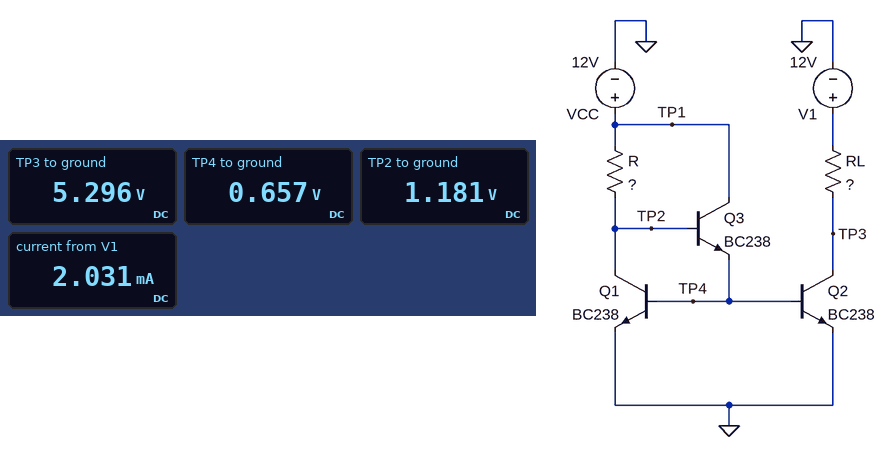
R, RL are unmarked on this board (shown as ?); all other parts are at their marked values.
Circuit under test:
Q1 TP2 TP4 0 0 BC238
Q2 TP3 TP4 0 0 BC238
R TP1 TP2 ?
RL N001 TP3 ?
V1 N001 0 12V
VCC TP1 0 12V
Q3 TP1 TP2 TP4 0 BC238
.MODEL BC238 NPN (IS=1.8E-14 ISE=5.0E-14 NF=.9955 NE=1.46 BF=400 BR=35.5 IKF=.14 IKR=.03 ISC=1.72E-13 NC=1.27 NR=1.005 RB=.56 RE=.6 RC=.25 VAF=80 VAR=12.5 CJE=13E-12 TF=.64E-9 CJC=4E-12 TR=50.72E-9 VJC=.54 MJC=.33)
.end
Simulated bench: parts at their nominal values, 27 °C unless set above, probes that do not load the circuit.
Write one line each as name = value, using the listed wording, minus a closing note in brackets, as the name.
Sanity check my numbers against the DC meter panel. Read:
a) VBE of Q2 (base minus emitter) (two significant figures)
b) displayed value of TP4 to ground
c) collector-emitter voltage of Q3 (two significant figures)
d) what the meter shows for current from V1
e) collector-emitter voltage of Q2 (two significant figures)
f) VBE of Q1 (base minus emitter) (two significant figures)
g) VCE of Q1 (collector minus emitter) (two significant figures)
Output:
VBE of Q2 (base minus emitter) = 660 mV
displayed value of TP4 to ground = 0.657 V
collector-emitter voltage of Q3 = 11 V
what the meter shows for current from V1 = 2.031 mA
collector-emitter voltage of Q2 = 5.3 V
VBE of Q1 (base minus emitter) = 660 mV
VCE of Q1 (collector minus emitter) = 1.2 V
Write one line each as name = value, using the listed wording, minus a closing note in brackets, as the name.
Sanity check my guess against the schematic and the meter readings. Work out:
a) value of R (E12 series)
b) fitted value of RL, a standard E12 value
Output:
value of R = 5.6 kΩ
fitted value of RL, a standard E12 value = 3.3 kΩ
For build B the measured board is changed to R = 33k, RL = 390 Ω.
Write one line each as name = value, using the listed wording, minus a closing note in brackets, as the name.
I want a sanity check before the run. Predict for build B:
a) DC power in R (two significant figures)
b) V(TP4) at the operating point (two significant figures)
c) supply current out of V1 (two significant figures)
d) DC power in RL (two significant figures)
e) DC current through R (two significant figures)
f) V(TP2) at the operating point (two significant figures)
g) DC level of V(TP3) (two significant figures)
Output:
DC power in R = 3.6 mW
V(TP4) at the operating point = 610 mV
supply current out of V1 = 380 µA
DC power in RL = 55 µW
DC current through R = 330 µA
V(TP2) at the operating point = 1.1 V
DC level of V(TP3) = 12 V
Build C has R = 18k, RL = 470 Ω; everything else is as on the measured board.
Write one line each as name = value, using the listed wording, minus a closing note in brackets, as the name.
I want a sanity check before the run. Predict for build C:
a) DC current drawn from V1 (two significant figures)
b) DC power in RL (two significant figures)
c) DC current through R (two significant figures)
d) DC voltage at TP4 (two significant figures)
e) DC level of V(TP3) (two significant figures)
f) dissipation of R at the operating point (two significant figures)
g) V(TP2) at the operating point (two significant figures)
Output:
DC current drawn from V1 = 690 µA
DC power in RL = 220 µW
DC current through R = 600 µA
DC voltage at TP4 = 630 mV
DC level of V(TP3) = 12 V
dissipation of R at the operating point = 6.6 mW
V(TP2) at the operating point = 1.1 V
